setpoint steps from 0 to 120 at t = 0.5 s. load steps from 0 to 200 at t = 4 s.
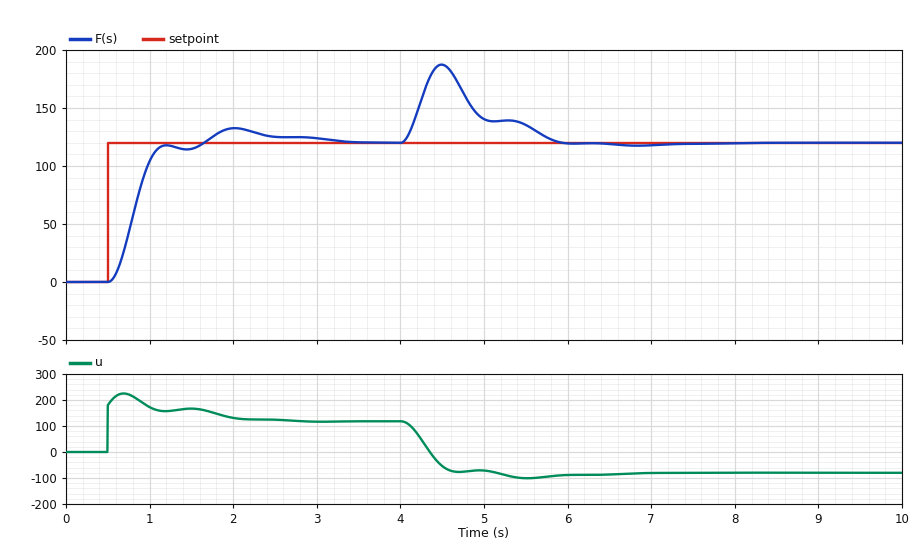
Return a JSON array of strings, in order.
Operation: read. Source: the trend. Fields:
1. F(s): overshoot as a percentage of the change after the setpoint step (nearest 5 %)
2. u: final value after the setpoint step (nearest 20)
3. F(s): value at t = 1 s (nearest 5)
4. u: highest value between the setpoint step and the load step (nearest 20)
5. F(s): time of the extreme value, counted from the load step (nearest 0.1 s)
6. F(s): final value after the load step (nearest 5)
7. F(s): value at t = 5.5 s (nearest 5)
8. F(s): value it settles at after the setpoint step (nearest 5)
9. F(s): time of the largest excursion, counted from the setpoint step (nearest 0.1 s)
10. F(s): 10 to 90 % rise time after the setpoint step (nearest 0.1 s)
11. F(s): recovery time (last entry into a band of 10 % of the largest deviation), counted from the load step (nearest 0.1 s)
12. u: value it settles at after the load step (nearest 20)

["10 %", "120", "105", "220", "0.5 s", "120", "135", "120", "1.5 s", "0.4 s", "1.7 s", "-80"]
